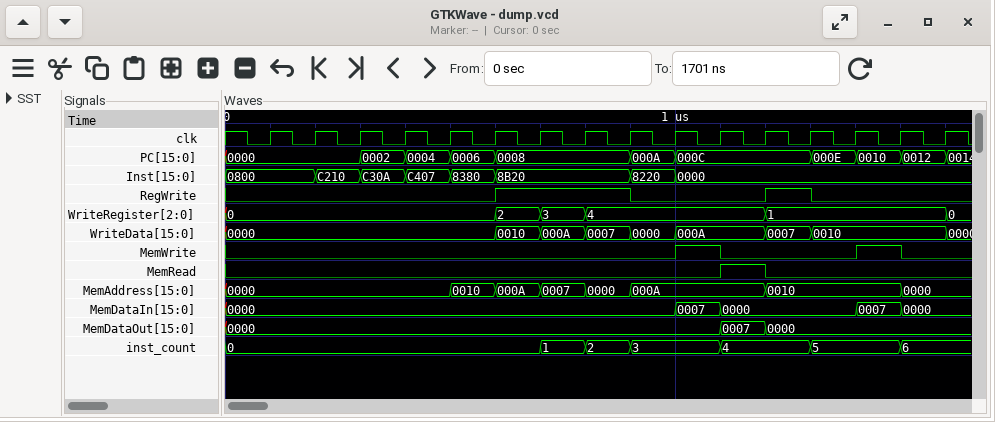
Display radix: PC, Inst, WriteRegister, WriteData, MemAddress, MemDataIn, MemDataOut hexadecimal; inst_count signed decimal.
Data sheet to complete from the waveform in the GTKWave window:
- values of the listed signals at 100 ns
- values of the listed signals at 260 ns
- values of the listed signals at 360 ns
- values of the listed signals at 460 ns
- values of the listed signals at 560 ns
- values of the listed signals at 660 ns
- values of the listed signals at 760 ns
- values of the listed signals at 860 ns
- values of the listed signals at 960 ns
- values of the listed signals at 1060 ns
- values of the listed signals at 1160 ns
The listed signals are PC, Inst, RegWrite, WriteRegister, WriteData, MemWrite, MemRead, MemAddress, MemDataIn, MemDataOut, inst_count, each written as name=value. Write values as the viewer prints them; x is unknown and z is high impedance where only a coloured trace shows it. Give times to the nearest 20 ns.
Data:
PC=0000, Inst=0800, RegWrite=0, WriteRegister=0, WriteData=0000, MemWrite=0, MemRead=0, MemAddress=0000, MemDataIn=0000, MemDataOut=0000, inst_count=0
PC=0000, Inst=C210, RegWrite=0, WriteRegister=0, WriteData=0000, MemWrite=0, MemRead=0, MemAddress=0000, MemDataIn=0000, MemDataOut=0000, inst_count=0
PC=0002, Inst=C30A, RegWrite=0, WriteRegister=0, WriteData=0000, MemWrite=0, MemRead=0, MemAddress=0000, MemDataIn=0000, MemDataOut=0000, inst_count=0
PC=0004, Inst=C407, RegWrite=0, WriteRegister=0, WriteData=0000, MemWrite=0, MemRead=0, MemAddress=0000, MemDataIn=0000, MemDataOut=0000, inst_count=0
PC=0006, Inst=8380, RegWrite=0, WriteRegister=0, WriteData=0000, MemWrite=0, MemRead=0, MemAddress=0010, MemDataIn=0000, MemDataOut=0000, inst_count=0
PC=0008, Inst=8B20, RegWrite=1, WriteRegister=2, WriteData=0010, MemWrite=0, MemRead=0, MemAddress=000A, MemDataIn=0000, MemDataOut=0000, inst_count=0
PC=0008, Inst=8B20, RegWrite=1, WriteRegister=3, WriteData=000A, MemWrite=0, MemRead=0, MemAddress=0007, MemDataIn=0000, MemDataOut=0000, inst_count=1
PC=0008, Inst=8B20, RegWrite=1, WriteRegister=4, WriteData=0007, MemWrite=0, MemRead=0, MemAddress=0000, MemDataIn=0000, MemDataOut=0000, inst_count=2
PC=000A, Inst=8220, RegWrite=0, WriteRegister=4, WriteData=0000, MemWrite=0, MemRead=0, MemAddress=000A, MemDataIn=0000, MemDataOut=0000, inst_count=3
PC=000C, Inst=0000, RegWrite=0, WriteRegister=4, WriteData=000A, MemWrite=1, MemRead=0, MemAddress=000A, MemDataIn=0007, MemDataOut=0000, inst_count=3
PC=000C, Inst=0000, RegWrite=0, WriteRegister=4, WriteData=000A, MemWrite=0, MemRead=1, MemAddress=000A, MemDataIn=0000, MemDataOut=0007, inst_count=4
